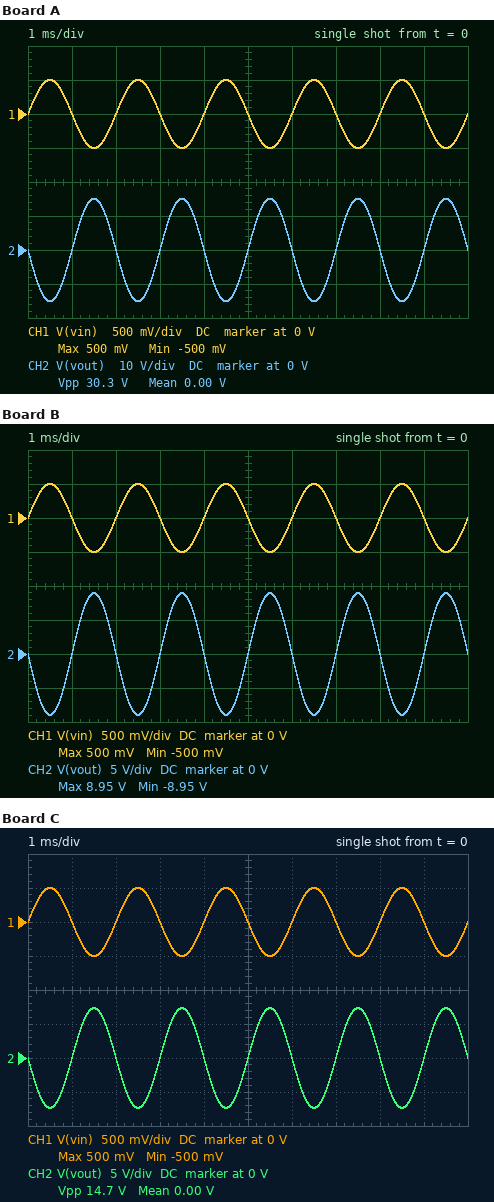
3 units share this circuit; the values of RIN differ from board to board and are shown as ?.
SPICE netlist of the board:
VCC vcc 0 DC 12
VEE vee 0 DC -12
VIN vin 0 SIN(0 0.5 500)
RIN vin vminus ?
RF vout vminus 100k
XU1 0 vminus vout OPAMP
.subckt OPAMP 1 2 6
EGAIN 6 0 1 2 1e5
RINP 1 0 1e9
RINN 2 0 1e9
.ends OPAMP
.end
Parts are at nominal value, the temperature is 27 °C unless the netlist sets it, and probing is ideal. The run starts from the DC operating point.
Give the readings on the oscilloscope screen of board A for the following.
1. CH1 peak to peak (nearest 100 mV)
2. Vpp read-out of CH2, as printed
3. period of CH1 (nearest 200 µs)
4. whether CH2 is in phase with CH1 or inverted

1.0 V
30.3 V
2.0 ms
inverted
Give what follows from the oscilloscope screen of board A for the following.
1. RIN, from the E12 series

3.3 kΩ
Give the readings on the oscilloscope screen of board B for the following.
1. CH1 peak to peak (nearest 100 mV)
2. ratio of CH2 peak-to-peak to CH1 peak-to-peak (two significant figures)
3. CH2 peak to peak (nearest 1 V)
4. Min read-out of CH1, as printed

1.0 V
18
18 V
-500 mV
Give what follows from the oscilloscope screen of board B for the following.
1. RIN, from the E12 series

5.6 kΩ
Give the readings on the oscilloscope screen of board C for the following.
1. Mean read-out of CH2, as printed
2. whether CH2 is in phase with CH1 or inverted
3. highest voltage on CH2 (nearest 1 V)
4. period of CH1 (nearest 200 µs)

0.00 V
inverted
7 V
2.0 ms
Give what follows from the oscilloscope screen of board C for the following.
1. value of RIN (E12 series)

6.8 kΩ
